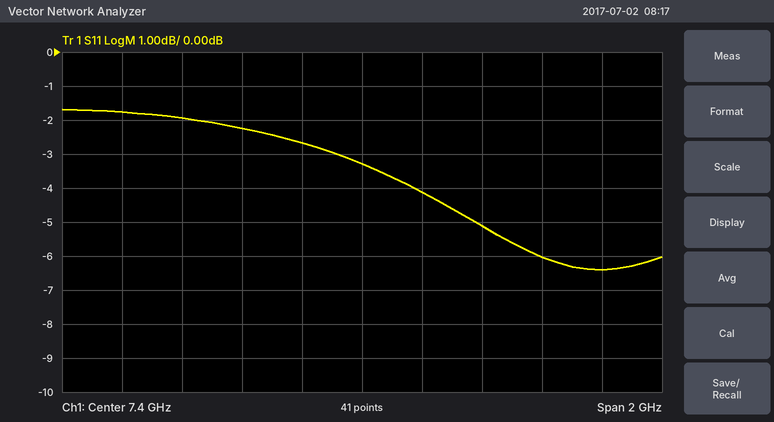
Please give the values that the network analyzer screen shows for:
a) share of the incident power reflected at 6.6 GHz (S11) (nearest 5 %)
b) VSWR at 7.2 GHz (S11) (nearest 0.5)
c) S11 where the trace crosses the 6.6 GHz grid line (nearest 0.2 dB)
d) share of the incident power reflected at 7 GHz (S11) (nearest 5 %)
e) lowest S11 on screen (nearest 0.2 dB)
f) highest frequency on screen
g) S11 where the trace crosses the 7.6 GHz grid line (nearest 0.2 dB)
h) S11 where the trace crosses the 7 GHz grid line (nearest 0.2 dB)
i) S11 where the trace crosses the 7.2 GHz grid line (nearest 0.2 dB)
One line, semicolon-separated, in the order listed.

65 %; 6.5; -1.8 dB; 60 %; -6.4 dB; 8.4 GHz; -4.2 dB; -2.2 dB; -2.6 dB
